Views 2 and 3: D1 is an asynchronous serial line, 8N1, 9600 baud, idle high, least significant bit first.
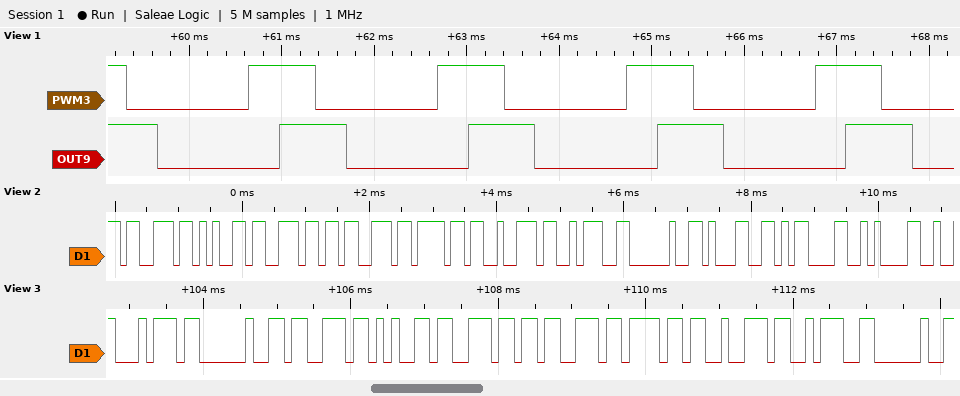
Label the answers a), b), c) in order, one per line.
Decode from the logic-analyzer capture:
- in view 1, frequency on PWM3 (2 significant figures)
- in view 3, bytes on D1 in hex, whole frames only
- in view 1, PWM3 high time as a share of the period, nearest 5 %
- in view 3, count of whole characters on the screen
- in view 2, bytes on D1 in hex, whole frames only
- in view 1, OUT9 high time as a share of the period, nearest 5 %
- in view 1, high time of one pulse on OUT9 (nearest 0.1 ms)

a) 490 Hz
b) 74 20 73 65 6E 73 6F 72 3A 20
c) 35 %
d) 10
e) 73 65 6E 73 6F 72 3A 20 31 0D 0A
f) 35 %
g) 0.7 ms
